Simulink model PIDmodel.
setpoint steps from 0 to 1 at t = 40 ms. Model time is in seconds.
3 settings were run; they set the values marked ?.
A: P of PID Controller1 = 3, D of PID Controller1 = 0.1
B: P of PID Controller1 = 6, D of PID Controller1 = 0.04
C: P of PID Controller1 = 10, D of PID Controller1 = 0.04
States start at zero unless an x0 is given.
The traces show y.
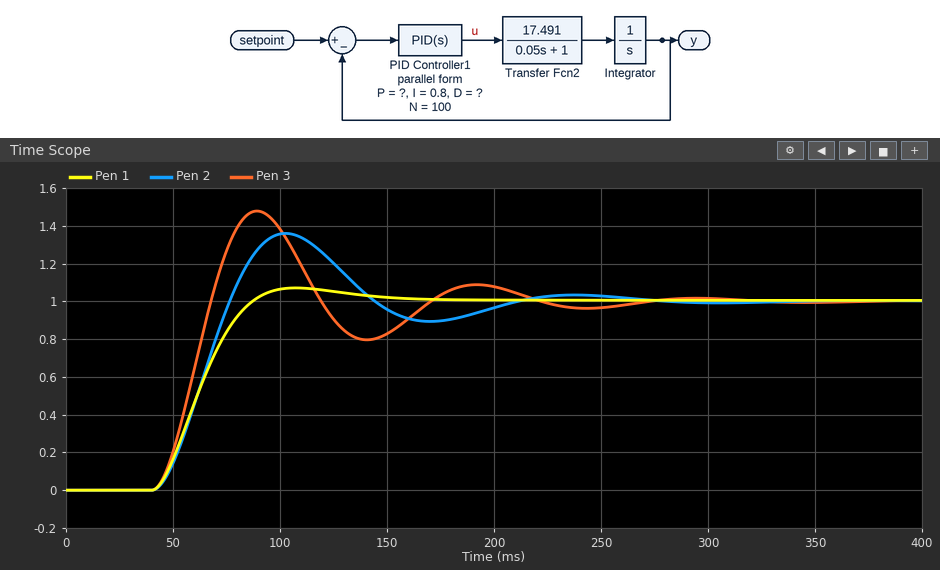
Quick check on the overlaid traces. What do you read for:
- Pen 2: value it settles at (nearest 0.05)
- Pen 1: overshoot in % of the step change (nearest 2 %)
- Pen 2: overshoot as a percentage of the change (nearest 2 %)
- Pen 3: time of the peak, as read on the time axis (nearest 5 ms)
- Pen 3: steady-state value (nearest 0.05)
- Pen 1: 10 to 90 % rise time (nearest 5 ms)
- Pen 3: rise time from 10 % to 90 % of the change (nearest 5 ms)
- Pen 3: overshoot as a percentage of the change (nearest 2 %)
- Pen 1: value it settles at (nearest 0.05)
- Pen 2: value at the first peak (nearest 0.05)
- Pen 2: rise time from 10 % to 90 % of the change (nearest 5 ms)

1.00
6 %
36 %
90 ms
1.00
30 ms
20 ms
48 %
1.00
1.35
25 ms
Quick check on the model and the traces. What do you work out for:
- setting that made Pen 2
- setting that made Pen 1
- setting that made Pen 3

B
A
C
